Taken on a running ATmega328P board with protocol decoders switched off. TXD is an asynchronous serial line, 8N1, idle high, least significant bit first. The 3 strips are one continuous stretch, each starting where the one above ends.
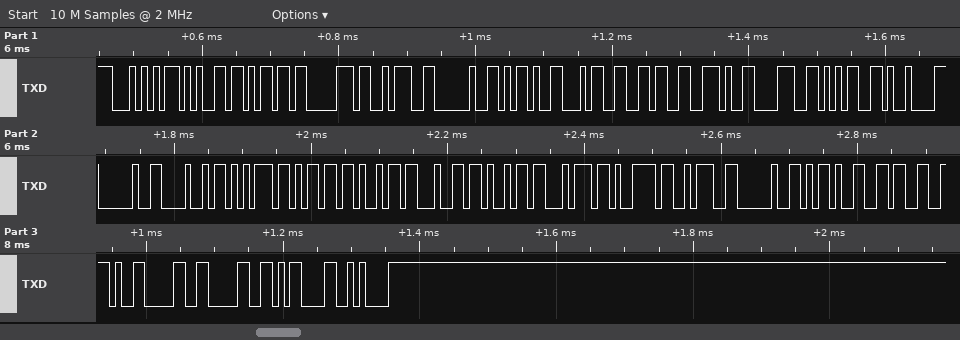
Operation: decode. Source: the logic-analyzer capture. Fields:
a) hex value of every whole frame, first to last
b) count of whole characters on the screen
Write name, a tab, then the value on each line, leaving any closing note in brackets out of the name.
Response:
hex value of every whole frame, first to last	54 65 6D 70 3A 20 2D 34 36 2E 38 35 09 20 48 75 6D 69 64 69 74 79 3A 20 2D 36 2E 30 30 0D 0A
count of whole characters on the screen	31
